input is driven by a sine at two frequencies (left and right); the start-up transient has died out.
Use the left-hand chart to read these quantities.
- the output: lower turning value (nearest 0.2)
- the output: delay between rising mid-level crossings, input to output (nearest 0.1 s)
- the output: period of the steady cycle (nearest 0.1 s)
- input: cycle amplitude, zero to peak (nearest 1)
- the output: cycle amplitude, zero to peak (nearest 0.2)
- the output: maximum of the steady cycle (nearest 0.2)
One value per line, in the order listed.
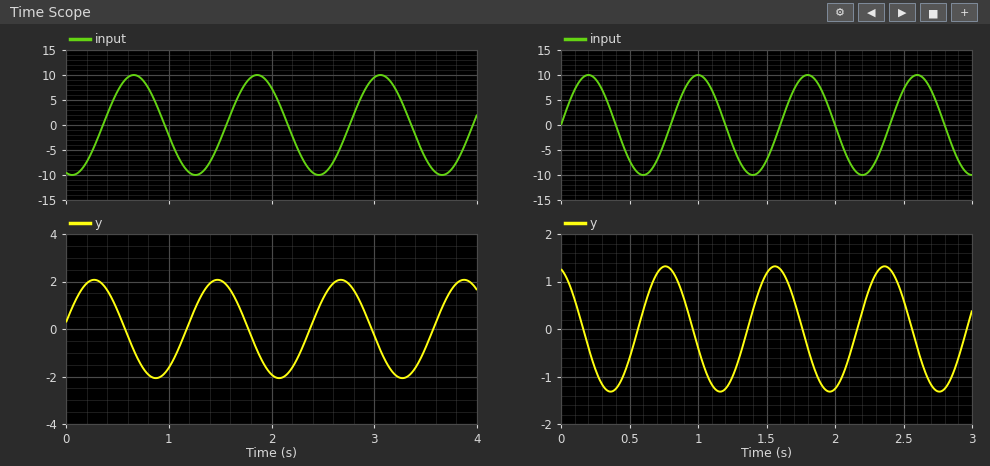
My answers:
-2.0
0.8 s
1.2 s
10
2.0
2.0
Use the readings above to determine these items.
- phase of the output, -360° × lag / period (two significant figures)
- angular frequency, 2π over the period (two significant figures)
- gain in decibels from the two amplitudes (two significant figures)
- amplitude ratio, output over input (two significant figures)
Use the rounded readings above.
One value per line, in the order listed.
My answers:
-240°
5.2 rad/s
-14 dB
0.20
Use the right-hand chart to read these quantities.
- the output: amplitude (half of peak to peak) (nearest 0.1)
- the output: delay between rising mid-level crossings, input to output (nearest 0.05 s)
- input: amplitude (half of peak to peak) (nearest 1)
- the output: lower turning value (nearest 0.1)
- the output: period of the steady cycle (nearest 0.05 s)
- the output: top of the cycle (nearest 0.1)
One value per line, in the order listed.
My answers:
1.3
0.55 s
10
-1.3
0.80 s
1.3
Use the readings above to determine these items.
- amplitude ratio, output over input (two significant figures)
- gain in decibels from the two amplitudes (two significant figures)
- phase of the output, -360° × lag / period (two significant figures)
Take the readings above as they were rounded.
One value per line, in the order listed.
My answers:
0.13
-18 dB
-250°
